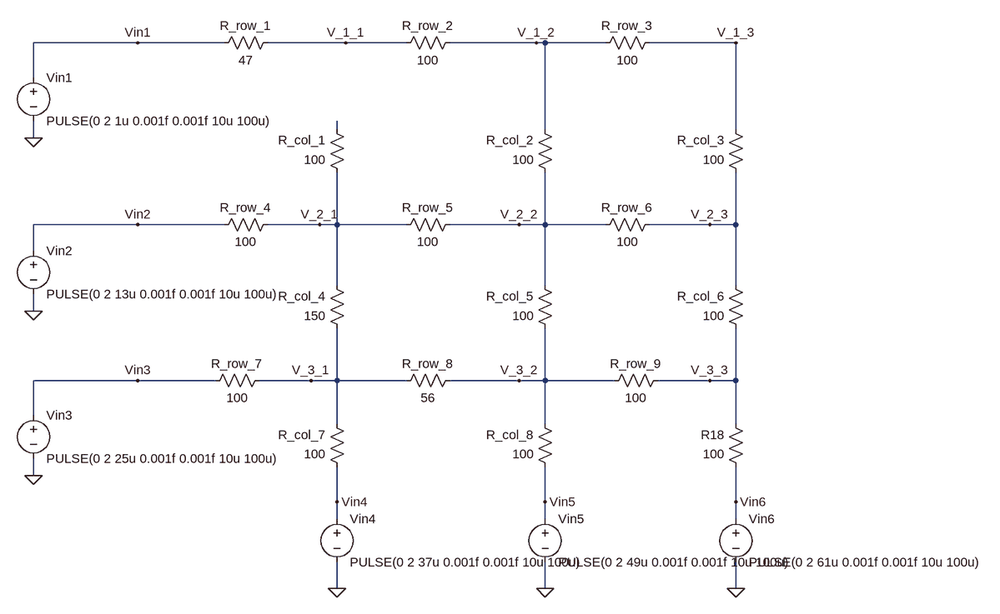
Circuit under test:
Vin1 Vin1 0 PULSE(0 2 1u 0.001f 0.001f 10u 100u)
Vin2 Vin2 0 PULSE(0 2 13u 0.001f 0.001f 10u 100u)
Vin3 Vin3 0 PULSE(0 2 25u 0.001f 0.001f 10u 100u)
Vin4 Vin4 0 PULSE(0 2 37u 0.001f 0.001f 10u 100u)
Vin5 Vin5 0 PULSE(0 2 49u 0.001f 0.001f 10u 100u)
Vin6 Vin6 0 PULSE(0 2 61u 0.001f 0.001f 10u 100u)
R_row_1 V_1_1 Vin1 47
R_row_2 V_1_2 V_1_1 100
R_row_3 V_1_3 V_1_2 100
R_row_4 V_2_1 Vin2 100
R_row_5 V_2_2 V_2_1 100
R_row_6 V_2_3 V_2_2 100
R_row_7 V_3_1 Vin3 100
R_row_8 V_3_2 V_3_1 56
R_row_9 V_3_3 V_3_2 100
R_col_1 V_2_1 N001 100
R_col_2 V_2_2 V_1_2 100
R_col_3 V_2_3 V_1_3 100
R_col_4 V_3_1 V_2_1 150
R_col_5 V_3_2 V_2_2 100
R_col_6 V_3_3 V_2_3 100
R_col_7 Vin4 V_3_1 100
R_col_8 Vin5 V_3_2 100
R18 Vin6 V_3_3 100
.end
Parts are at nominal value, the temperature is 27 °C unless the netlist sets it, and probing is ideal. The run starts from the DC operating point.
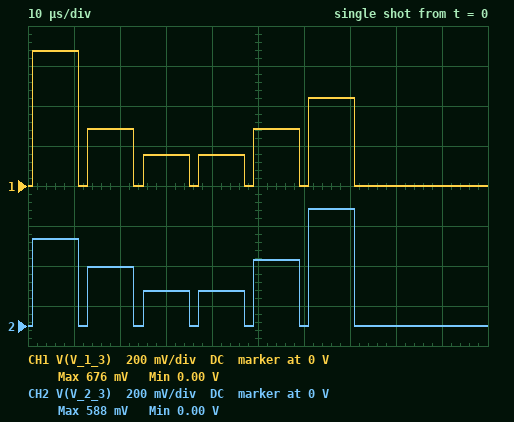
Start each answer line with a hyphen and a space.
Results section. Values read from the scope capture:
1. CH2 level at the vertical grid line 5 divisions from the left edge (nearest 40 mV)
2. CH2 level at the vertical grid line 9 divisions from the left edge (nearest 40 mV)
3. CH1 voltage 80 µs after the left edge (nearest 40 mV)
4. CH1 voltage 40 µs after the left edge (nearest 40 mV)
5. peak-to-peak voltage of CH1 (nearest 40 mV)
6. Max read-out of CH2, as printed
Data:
- 320 mV
- 0 V
- 0 V
- 160 mV
- 680 mV
- 588 mV
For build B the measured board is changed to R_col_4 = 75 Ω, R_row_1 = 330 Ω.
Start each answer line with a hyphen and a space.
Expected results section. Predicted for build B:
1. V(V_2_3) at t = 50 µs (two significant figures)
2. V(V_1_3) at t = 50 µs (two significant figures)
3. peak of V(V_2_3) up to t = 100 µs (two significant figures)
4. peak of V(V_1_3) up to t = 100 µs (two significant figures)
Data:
- 380 mV
- 370 mV
- 650 mV
- 530 mV
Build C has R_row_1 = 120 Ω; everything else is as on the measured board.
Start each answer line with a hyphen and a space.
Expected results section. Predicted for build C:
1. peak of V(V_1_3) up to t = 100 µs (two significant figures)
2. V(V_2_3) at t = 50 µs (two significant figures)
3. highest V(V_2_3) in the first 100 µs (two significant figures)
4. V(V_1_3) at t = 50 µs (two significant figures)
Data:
- 530 mV
- 350 mV
- 610 mV
- 320 mV
